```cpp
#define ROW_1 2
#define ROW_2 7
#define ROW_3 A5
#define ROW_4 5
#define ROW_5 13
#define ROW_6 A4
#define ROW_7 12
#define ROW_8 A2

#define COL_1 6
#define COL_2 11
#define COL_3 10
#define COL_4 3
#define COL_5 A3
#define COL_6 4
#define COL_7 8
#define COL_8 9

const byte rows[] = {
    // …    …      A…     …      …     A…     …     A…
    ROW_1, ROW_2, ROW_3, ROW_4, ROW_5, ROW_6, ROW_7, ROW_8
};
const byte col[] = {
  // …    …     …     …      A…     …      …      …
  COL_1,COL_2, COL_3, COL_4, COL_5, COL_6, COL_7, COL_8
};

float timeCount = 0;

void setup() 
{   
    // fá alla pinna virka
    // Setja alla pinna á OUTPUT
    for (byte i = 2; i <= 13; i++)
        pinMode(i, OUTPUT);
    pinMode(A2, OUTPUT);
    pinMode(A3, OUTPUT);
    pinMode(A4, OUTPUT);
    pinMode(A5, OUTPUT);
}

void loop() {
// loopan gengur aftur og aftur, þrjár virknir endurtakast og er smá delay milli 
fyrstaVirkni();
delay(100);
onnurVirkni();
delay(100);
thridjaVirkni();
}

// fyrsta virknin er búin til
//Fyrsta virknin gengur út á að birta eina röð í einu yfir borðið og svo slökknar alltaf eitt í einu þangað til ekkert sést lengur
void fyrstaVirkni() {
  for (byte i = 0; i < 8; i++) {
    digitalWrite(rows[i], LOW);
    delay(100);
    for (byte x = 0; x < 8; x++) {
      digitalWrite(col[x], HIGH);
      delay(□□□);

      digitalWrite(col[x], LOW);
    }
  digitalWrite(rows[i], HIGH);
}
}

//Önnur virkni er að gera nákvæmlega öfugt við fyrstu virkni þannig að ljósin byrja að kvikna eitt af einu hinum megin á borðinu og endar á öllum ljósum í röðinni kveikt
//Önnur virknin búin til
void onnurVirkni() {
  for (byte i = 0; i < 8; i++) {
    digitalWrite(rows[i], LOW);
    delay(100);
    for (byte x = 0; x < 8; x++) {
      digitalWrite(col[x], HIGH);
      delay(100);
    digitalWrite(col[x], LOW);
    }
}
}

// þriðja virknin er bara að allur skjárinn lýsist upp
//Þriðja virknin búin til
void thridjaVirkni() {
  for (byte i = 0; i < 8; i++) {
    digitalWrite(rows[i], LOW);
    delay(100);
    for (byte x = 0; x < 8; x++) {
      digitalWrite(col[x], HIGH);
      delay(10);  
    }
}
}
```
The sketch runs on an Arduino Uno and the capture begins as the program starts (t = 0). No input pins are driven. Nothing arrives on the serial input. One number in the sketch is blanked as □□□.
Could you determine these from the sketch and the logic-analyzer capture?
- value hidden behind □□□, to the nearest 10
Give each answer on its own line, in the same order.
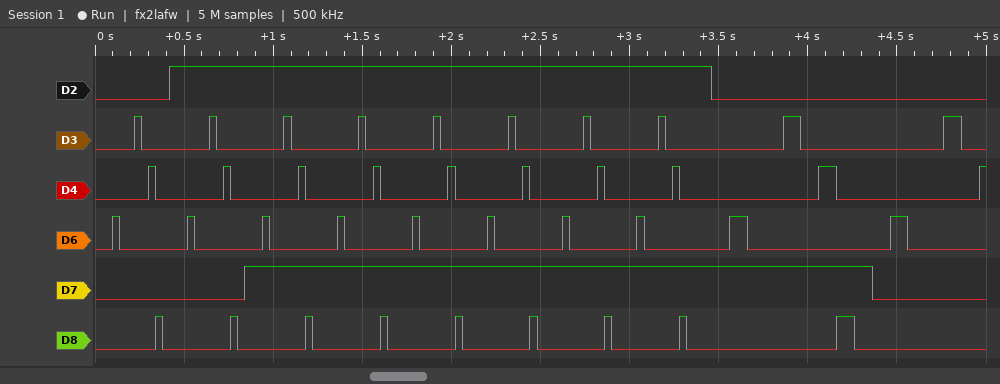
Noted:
40
